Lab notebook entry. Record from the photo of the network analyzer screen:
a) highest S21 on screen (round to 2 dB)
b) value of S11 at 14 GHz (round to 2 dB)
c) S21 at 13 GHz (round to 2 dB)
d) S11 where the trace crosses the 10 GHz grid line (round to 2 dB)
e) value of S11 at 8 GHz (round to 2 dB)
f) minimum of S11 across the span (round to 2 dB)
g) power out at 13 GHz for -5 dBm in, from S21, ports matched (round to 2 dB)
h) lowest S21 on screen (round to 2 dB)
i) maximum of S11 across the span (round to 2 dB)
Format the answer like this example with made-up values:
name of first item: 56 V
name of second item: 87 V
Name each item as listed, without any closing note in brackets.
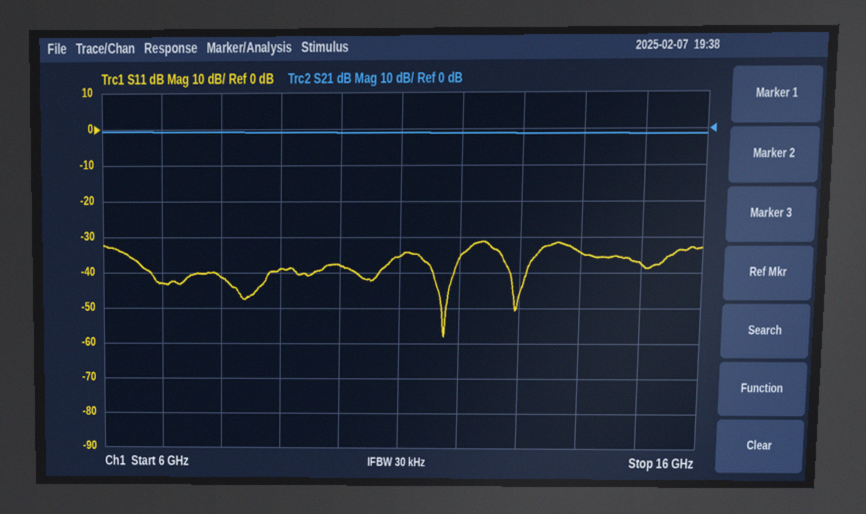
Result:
highest S21 on screen: 0 dB
value of S11 at 14 GHz: -34 dB
S21 at 13 GHz: -2 dB
S11 where the trace crosses the 10 GHz grid line: -38 dB
value of S11 at 8 GHz: -42 dB
minimum of S11 across the span: -58 dB
power out at 13 GHz for -5 dBm in, from S21, ports matched: -6 dBm
lowest S21 on screen: -2 dB
maximum of S11 across the span: -32 dB
